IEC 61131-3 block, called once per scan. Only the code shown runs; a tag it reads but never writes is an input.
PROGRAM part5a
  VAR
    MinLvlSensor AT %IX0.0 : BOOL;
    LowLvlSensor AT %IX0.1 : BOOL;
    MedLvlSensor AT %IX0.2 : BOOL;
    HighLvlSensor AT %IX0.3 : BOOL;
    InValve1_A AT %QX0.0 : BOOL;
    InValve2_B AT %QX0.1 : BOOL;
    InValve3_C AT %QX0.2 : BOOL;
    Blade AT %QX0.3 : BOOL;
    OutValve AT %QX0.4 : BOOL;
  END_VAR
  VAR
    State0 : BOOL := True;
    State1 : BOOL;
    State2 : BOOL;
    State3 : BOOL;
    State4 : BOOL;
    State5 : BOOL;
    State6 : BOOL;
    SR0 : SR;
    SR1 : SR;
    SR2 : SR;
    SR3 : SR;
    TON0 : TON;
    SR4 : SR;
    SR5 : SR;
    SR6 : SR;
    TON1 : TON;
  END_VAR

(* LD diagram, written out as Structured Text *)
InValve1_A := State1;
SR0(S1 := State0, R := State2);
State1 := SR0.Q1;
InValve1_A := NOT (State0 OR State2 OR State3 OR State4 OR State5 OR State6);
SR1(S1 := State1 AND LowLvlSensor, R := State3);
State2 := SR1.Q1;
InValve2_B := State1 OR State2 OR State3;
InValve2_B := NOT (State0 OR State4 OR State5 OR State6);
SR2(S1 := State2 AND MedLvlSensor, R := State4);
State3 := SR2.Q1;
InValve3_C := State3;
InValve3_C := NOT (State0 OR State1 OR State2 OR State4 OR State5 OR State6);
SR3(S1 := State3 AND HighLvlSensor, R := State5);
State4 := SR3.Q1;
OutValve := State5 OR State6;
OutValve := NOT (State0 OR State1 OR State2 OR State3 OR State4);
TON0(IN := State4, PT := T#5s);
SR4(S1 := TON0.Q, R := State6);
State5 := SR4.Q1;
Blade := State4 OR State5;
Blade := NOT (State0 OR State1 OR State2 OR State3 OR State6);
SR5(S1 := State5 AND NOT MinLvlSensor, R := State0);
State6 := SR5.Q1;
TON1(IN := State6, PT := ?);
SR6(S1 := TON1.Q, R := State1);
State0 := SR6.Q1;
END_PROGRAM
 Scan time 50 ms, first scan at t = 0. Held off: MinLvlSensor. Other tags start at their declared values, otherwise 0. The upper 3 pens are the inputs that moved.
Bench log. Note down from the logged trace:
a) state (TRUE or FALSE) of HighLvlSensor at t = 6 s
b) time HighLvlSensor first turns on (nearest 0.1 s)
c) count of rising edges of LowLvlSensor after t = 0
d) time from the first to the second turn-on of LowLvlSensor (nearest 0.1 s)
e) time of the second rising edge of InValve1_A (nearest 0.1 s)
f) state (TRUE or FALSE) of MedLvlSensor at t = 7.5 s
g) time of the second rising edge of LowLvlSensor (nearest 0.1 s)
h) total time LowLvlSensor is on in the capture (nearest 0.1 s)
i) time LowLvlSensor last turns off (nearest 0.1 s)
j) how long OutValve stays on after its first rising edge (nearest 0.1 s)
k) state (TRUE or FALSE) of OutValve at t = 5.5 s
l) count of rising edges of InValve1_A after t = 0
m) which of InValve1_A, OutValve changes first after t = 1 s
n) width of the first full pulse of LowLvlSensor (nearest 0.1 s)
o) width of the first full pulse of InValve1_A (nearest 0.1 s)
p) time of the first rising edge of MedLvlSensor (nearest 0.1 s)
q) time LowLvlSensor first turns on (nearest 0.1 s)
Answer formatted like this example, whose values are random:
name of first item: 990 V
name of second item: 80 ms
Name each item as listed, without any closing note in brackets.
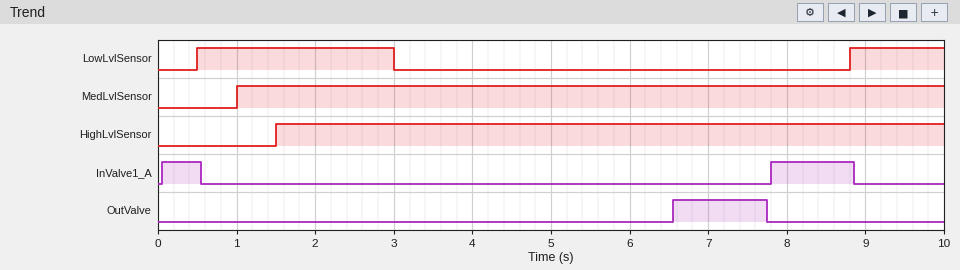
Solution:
state (TRUE or FALSE) of HighLvlSensor at t = 6 s: TRUE
time HighLvlSensor first turns on: 1.5 s
count of rising edges of LowLvlSensor after t = 0: 2
time from the first to the second turn-on of LowLvlSensor: 8.3 s
time of the second rising edge of InValve1_A: 7.8 s
state (TRUE or FALSE) of MedLvlSensor at t = 7.5 s: TRUE
time of the second rising edge of LowLvlSensor: 8.8 s
total time LowLvlSensor is on in the capture: 3.7 s
time LowLvlSensor last turns off: 3.0 s
how long OutValve stays on after its first rising edge: 1.2 s
state (TRUE or FALSE) of OutValve at t = 5.5 s: FALSE
count of rising edges of InValve1_A after t = 0: 2
which of InValve1_A, OutValve changes first after t = 1 s: OutValve
width of the first full pulse of LowLvlSensor: 2.5 s
width of the first full pulse of InValve1_A: 0.5 s
time of the first rising edge of MedLvlSensor: 1.0 s
time LowLvlSensor first turns on: 0.5 s
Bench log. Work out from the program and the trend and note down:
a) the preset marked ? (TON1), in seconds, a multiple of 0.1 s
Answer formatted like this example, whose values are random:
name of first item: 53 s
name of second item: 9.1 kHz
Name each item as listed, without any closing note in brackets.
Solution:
the preset marked ? (TON1), in seconds, a multiple of 0.1 s: 1.2 s
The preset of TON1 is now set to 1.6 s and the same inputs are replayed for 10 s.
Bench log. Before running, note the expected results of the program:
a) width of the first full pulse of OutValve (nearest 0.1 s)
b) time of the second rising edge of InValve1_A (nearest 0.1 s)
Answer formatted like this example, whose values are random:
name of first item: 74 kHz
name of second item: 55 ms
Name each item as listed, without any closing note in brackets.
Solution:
width of the first full pulse of OutValve: 1.6 s
time of the second rising edge of InValve1_A: 8.2 s
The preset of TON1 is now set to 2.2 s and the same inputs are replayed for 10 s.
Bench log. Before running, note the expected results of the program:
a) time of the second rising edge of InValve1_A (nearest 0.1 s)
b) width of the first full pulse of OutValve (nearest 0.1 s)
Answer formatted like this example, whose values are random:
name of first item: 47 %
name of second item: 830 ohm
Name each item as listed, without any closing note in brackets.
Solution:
time of the second rising edge of InValve1_A: 8.8 s
width of the first full pulse of OutValve: 2.2 s
